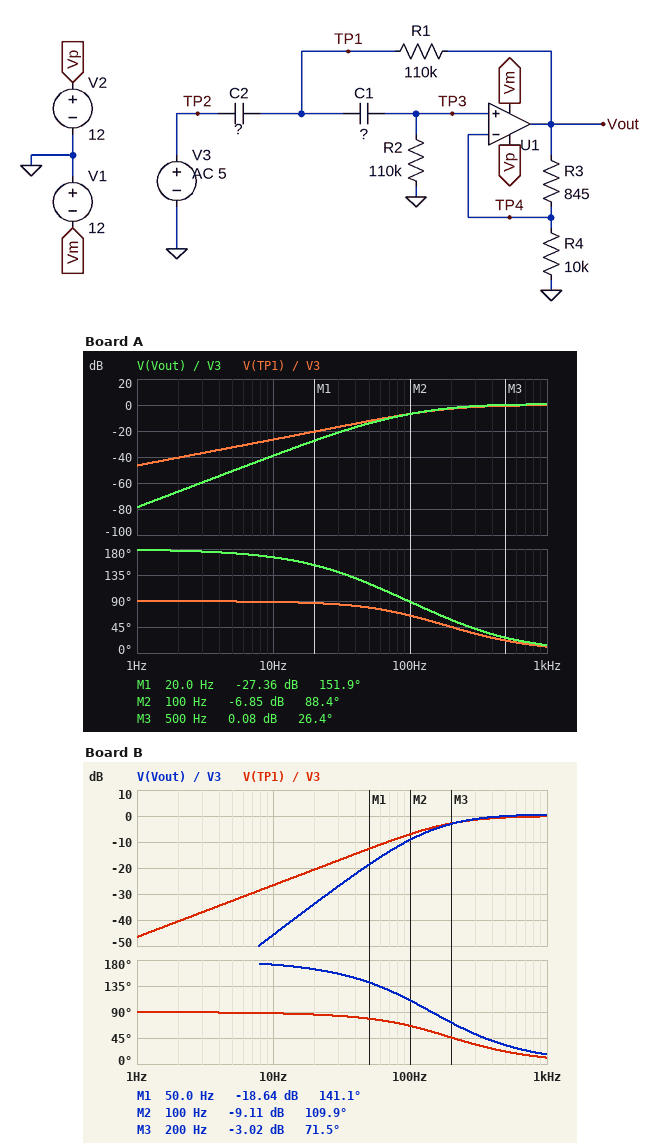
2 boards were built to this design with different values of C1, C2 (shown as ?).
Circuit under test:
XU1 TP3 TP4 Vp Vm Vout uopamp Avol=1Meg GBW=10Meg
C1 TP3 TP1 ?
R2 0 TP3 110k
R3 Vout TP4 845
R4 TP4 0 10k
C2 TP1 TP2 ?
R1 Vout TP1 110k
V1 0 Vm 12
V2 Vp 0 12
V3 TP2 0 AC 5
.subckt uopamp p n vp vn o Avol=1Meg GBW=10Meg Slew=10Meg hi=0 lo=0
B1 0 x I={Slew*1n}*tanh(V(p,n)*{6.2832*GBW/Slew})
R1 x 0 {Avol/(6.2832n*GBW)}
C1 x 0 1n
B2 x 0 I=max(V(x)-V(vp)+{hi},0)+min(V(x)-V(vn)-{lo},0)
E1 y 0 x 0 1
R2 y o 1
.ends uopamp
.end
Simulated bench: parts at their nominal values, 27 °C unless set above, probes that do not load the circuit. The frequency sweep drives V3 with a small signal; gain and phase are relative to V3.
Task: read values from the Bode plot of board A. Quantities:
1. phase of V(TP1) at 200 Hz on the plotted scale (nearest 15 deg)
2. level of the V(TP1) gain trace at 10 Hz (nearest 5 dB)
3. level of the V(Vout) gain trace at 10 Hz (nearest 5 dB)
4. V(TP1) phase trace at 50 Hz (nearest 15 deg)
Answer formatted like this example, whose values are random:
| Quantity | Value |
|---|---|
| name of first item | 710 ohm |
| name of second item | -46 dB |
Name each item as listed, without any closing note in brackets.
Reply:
| Quantity | Value |
|---|---|
| phase of V(TP1) at 200 Hz on the plotted scale | 45 deg |
| level of the V(TP1) gain trace at 10 Hz | -25 dB |
| level of the V(Vout) gain trace at 10 Hz | -40 dB |
| V(TP1) phase trace at 50 Hz | 75 deg |
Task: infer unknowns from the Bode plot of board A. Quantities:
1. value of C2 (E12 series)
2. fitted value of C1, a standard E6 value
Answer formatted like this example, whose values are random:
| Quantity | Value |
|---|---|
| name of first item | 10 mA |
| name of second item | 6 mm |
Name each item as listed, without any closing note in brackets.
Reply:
| Quantity | Value |
|---|---|
| value of C2 | 6.8 nF |
| fitted value of C1, a standard E6 value | 33 nF |
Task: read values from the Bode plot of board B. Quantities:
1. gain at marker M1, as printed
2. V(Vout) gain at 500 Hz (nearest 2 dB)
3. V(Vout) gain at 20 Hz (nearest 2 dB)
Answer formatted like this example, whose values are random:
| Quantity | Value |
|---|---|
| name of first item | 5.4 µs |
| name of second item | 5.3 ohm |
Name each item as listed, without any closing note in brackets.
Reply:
| Quantity | Value |
|---|---|
| gain at marker M1, as printed | -18.64 dB |
| V(Vout) gain at 500 Hz | 0 dB |
| V(Vout) gain at 20 Hz | -34 dB |
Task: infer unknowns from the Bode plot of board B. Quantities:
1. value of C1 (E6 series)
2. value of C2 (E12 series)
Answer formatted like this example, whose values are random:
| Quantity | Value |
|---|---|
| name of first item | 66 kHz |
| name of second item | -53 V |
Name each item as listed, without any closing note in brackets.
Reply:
| Quantity | Value |
|---|---|
| value of C1 | 15 nF |
| value of C2 | 6.8 nF |
